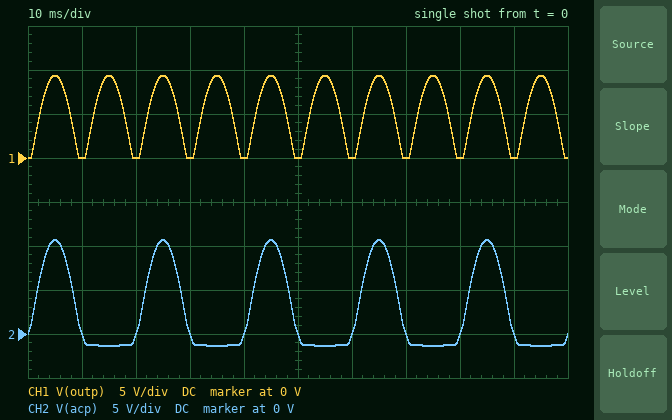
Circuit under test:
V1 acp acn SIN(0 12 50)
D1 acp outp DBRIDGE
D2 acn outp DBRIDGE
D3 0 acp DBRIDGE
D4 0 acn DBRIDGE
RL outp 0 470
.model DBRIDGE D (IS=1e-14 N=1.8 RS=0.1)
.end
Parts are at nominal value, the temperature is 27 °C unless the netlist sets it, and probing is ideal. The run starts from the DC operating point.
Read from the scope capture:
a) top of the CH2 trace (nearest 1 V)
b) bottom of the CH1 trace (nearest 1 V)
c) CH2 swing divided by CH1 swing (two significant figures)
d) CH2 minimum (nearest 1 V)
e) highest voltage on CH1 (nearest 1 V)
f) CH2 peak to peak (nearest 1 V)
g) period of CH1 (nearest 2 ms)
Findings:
11 V
0 V
1.3
-1 V
9 V
12 V
10 ms
